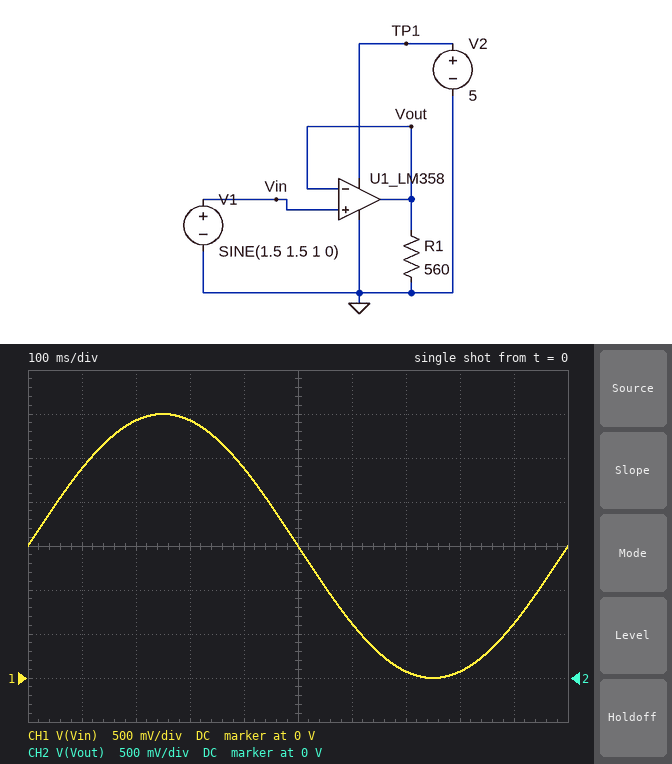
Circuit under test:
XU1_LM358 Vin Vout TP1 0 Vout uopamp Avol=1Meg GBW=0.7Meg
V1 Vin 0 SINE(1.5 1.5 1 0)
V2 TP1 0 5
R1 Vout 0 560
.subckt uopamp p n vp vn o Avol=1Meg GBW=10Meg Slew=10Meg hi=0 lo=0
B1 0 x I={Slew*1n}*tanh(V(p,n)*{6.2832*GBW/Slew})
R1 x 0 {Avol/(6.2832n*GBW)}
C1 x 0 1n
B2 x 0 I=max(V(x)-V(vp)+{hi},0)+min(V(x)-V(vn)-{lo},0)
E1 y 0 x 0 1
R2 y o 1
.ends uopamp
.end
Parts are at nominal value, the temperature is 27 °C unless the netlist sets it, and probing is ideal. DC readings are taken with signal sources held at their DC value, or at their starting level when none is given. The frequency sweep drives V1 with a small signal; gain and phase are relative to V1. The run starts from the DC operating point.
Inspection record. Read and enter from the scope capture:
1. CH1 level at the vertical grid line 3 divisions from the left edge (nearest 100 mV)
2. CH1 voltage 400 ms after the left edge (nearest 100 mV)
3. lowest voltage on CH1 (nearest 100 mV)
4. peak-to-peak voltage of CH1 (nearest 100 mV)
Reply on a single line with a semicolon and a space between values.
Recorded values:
2.9 V; 2.4 V; 0 V; 3.0 V
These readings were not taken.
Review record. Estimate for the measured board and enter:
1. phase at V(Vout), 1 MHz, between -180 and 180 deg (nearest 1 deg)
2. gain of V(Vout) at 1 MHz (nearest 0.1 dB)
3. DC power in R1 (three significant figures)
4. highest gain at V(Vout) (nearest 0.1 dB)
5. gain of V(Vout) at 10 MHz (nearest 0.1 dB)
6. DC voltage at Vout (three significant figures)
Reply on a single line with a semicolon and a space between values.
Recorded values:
-55 deg; -4.8 dB; 4.02 mW; 0 dB; -23.1 dB; 1.50 V
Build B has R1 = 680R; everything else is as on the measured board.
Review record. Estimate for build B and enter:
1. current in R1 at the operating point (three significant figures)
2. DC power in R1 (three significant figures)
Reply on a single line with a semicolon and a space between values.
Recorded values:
2.21 mA; 3.31 mW
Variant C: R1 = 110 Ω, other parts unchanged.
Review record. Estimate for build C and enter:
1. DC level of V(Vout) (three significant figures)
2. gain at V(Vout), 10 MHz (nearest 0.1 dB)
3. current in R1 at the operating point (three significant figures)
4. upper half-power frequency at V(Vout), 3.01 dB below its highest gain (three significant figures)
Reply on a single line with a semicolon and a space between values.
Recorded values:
1.50 V; -23.2 dB; 13.6 mA; 694 kHz
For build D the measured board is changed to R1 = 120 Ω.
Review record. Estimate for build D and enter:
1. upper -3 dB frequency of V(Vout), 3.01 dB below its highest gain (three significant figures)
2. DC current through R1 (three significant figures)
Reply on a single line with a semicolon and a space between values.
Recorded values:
694 kHz; 12.5 mA
